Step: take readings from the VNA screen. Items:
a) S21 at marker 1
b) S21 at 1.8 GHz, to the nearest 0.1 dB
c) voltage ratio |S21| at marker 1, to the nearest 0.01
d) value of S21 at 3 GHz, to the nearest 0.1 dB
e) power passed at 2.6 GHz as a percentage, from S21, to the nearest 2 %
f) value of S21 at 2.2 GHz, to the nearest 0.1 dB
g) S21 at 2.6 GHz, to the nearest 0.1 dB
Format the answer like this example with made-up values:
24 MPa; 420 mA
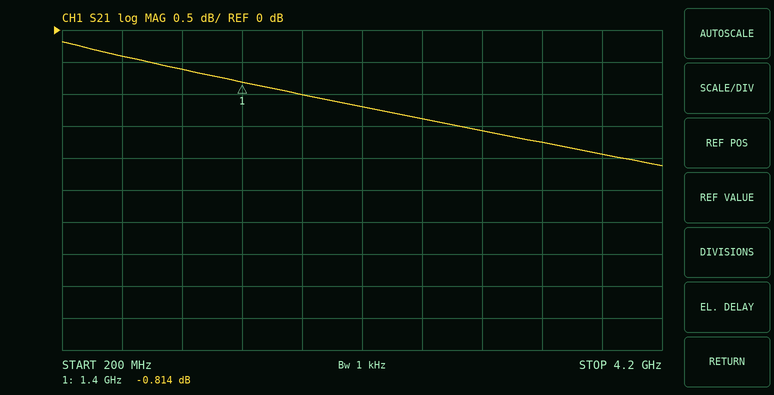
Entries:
-0.814 dB; -1.0 dB; 0.91; -1.6 dB; 72 %; -1.2 dB; -1.4 dB
